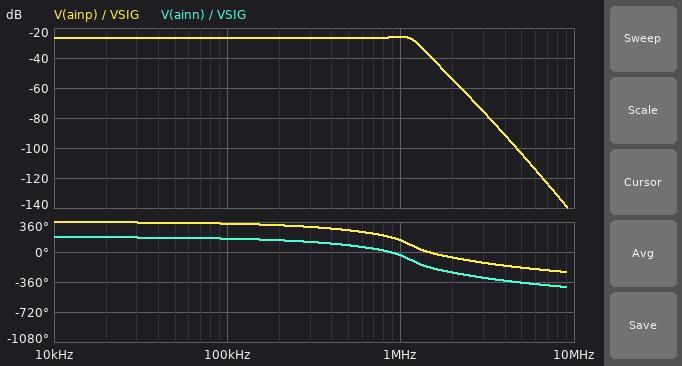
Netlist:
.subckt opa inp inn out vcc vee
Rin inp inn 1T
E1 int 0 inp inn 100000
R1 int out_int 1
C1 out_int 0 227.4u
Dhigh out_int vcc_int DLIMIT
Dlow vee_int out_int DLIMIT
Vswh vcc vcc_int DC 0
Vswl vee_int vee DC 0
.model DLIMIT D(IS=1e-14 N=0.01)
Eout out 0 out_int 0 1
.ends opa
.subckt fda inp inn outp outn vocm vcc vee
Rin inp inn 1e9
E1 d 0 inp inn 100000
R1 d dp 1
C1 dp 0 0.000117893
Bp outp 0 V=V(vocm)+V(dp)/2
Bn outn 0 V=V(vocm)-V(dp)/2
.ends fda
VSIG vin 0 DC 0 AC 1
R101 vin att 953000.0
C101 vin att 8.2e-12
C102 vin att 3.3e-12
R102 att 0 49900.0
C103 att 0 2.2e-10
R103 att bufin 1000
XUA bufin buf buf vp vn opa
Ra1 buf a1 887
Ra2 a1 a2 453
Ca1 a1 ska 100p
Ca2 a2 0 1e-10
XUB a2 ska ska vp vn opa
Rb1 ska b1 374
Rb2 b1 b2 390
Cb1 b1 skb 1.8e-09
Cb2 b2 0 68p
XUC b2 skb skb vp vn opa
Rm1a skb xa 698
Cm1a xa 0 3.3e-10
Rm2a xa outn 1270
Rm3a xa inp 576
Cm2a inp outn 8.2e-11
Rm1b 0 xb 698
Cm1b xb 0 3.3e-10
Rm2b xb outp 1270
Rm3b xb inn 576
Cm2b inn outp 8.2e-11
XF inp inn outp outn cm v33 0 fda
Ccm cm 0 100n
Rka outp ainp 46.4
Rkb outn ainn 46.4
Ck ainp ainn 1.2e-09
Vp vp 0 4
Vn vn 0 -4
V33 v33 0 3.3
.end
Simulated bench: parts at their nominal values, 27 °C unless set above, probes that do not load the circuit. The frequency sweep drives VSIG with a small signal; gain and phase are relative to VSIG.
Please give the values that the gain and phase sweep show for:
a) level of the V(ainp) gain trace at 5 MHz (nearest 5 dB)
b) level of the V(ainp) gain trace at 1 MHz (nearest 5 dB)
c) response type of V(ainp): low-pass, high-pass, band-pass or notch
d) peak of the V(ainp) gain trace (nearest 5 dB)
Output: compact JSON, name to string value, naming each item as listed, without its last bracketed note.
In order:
{"level of the V(ainp) gain trace at 5 MHz": "-105 dB", "level of the V(ainp) gain trace at 1 MHz": "-25 dB", "response type of V(ainp): low-pass, high-pass, band-pass or notch": "low-pass", "peak of the V(ainp) gain trace": "-25 dB"}
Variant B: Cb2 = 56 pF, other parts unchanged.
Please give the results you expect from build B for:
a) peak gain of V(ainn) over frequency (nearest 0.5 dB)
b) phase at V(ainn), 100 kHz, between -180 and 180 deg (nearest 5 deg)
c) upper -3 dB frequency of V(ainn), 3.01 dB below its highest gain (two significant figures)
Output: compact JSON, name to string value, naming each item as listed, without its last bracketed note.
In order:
{"peak gain of V(ainn) over frequency": "-26.5 dB", "phase at V(ainn), 100 kHz, between -180 and 180 deg": "160 deg", "upper -3 dB frequency of V(ainn), 3.01 dB below its highest gain": "1.3 MHz"}
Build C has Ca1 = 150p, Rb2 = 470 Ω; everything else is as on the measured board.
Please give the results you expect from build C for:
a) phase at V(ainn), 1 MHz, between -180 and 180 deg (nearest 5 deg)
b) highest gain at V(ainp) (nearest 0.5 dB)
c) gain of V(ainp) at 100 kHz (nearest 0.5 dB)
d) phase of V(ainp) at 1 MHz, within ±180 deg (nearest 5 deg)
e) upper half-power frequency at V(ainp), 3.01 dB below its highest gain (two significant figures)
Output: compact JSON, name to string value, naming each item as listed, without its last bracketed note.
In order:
{"phase at V(ainn), 1 MHz, between -180 and 180 deg": "-65 deg", "highest gain at V(ainp)": "-24.5 dB", "gain of V(ainp) at 100 kHz": "-27.0 dB", "phase of V(ainp) at 1 MHz, within ±180 deg": "115 deg", "upper half-power frequency at V(ainp), 3.01 dB below its highest gain": "1.1 MHz"}
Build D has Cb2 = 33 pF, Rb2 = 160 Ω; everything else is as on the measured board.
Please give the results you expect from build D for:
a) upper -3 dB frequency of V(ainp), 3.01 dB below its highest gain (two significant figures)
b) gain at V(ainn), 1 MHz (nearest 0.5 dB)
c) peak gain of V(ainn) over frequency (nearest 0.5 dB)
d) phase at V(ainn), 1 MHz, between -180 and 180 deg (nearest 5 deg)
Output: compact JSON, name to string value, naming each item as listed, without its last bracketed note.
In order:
{"upper -3 dB frequency of V(ainp), 3.01 dB below its highest gain": "760 kHz", "gain at V(ainn), 1 MHz": "-32.0 dB", "peak gain of V(ainn) over frequency": "-27.0 dB", "phase at V(ainn), 1 MHz, between -180 and 180 deg": "5 deg"}
